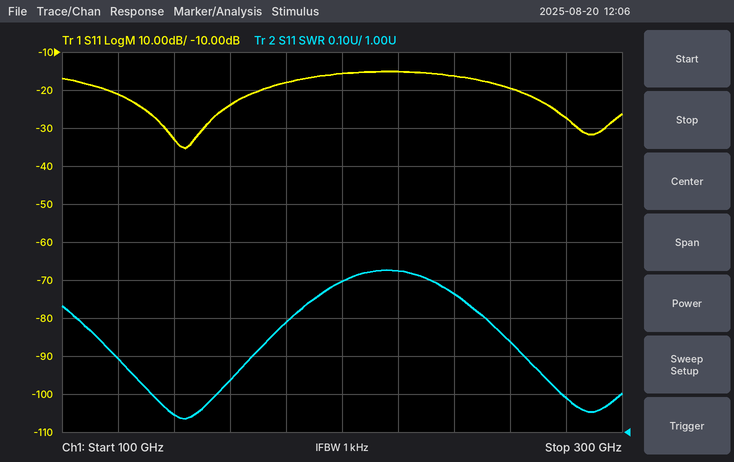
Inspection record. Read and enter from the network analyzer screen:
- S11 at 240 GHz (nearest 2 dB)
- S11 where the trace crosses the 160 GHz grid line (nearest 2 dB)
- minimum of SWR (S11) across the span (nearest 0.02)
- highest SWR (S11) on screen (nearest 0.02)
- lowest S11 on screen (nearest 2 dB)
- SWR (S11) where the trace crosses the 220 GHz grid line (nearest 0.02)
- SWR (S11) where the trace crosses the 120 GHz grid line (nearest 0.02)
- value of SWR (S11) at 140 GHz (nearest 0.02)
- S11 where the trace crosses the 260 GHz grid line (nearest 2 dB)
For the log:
-16 dB
-24 dB
1.04
1.42
-36 dB
1.42
1.20
1.04
-20 dB
